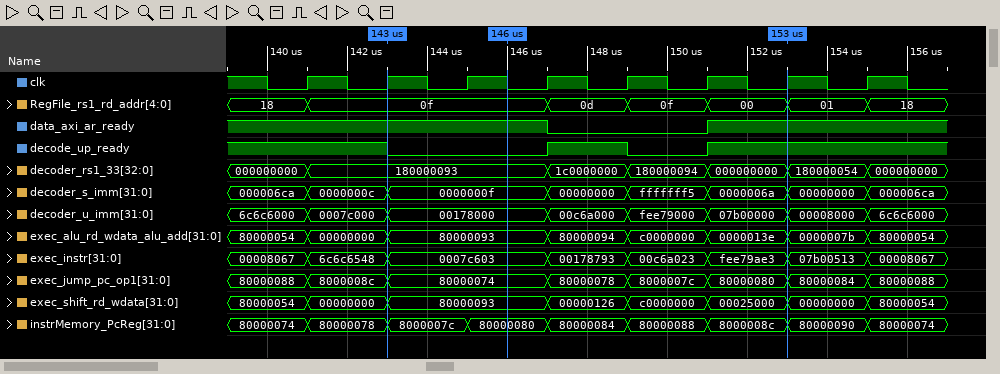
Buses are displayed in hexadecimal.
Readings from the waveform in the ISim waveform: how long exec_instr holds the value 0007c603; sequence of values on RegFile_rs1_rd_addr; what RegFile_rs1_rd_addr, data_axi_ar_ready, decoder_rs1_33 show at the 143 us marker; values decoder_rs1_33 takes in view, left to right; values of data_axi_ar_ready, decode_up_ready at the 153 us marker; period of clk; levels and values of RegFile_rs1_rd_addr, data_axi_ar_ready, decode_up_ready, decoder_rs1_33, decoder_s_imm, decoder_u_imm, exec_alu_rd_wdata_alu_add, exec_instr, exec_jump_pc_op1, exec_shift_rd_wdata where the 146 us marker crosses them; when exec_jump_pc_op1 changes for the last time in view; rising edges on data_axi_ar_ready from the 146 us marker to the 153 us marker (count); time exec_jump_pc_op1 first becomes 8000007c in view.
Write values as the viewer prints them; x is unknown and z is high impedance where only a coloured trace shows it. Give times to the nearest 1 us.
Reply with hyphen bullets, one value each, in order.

- 4 us
- 18, 0f, 0d, 0f, 00, 01, 18
- RegFile_rs1_rd_addr=0f, data_axi_ar_ready=1, decoder_rs1_33=180000093
- 000000000, 180000093, 1c0000000, 180000094, 000000000, 180000054, 000000000
- data_axi_ar_ready=1, decode_up_ready=1
- 2 us
- RegFile_rs1_rd_addr=0f, data_axi_ar_ready=1, decode_up_ready=0, decoder_rs1_33=180000093, decoder_s_imm=0000000f, decoder_u_imm=00178000, exec_alu_rd_wdata_alu_add=80000093, exec_instr=0007c603, exec_jump_pc_op1=80000074, exec_shift_rd_wdata=80000093
- 155 us
- 1
- 149 us
